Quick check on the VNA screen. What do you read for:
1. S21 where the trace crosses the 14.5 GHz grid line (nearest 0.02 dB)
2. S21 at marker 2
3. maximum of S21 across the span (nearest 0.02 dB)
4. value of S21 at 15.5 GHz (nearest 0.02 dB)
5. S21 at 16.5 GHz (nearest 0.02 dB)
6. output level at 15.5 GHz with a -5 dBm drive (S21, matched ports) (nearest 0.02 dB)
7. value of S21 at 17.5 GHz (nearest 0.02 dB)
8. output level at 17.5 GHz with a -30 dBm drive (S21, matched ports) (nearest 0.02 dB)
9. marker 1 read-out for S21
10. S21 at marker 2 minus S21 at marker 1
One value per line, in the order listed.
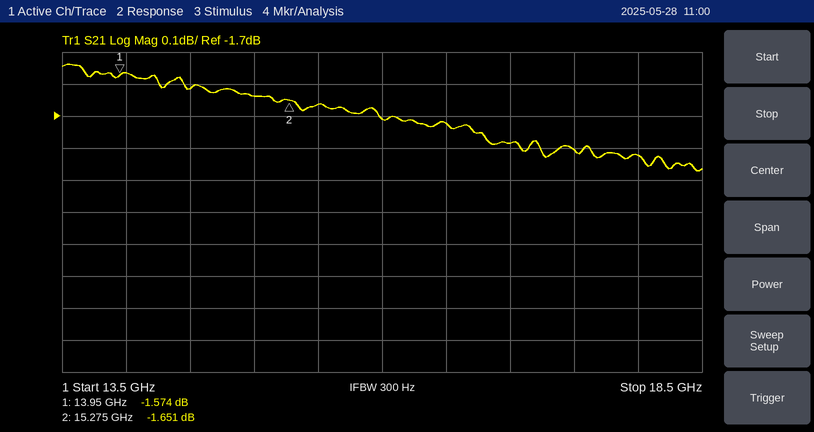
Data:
-1.62 dB
-1.651 dB
-1.54 dB
-1.66 dB
-1.72 dB
-6.66 dBm
-1.80 dB
-31.80 dBm
-1.574 dB
-0.077 dB
